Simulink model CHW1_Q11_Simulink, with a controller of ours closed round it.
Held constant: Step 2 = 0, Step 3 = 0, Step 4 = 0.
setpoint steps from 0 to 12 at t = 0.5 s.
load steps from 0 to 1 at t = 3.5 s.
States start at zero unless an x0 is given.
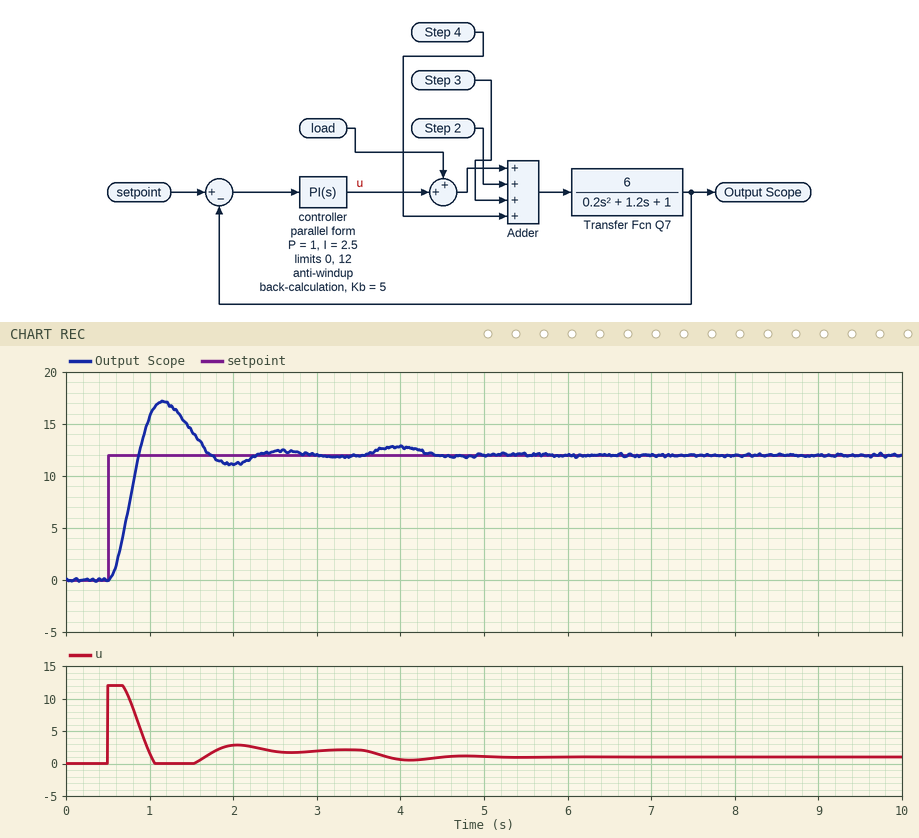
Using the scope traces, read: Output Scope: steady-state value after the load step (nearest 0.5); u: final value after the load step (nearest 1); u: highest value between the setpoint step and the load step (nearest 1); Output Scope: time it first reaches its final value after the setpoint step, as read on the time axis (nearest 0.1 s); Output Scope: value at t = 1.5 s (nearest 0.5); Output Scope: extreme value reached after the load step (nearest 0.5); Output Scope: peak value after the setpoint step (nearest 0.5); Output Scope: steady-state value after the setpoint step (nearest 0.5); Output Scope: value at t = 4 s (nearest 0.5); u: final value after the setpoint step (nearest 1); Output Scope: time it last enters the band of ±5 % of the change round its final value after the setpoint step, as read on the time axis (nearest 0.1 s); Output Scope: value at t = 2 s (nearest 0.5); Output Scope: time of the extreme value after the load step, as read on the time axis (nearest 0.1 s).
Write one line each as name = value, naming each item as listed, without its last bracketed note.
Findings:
Output Scope: steady-state value after the load step = 12.0
u: final value after the load step = 1
u: highest value between the setpoint step and the load step = 12
Output Scope: time it first reaches its final value after the setpoint step, as read on the time axis = 0.9 s
Output Scope: value at t = 1.5 s = 14.5
Output Scope: extreme value reached after the load step = 13.0
Output Scope: peak value after the setpoint step = 17.0
Output Scope: steady-state value after the setpoint step = 12.0
Output Scope: value at t = 4 s = 13.0
u: final value after the setpoint step = 2
Output Scope: time it last enters the band of ±5 % of the change round its final value after the setpoint step, as read on the time axis = 2.1 s
Output Scope: value at t = 2 s = 11.0
Output Scope: time of the extreme value after the load step, as read on the time axis = 4.0 s
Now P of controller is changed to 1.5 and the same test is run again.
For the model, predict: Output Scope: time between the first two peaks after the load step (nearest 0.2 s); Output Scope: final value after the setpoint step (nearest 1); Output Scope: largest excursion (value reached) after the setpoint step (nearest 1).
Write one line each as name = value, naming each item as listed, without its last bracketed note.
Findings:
Output Scope: time between the first two peaks after the load step = 1.0 s
Output Scope: final value after the setpoint step = 12
Output Scope: largest excursion (value reached) after the setpoint step = 15
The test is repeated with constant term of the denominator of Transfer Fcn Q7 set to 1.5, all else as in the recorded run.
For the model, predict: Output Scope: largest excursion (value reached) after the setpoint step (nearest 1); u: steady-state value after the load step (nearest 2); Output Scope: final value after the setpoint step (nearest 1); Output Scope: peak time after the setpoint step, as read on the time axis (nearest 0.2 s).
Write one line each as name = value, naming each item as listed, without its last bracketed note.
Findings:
Output Scope: largest excursion (value reached) after the setpoint step = 16
u: steady-state value after the load step = 2
Output Scope: final value after the setpoint step = 12
Output Scope: peak time after the setpoint step, as read on the time axis = 1.2 s
